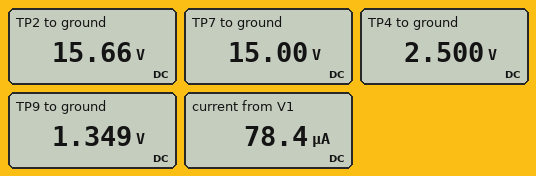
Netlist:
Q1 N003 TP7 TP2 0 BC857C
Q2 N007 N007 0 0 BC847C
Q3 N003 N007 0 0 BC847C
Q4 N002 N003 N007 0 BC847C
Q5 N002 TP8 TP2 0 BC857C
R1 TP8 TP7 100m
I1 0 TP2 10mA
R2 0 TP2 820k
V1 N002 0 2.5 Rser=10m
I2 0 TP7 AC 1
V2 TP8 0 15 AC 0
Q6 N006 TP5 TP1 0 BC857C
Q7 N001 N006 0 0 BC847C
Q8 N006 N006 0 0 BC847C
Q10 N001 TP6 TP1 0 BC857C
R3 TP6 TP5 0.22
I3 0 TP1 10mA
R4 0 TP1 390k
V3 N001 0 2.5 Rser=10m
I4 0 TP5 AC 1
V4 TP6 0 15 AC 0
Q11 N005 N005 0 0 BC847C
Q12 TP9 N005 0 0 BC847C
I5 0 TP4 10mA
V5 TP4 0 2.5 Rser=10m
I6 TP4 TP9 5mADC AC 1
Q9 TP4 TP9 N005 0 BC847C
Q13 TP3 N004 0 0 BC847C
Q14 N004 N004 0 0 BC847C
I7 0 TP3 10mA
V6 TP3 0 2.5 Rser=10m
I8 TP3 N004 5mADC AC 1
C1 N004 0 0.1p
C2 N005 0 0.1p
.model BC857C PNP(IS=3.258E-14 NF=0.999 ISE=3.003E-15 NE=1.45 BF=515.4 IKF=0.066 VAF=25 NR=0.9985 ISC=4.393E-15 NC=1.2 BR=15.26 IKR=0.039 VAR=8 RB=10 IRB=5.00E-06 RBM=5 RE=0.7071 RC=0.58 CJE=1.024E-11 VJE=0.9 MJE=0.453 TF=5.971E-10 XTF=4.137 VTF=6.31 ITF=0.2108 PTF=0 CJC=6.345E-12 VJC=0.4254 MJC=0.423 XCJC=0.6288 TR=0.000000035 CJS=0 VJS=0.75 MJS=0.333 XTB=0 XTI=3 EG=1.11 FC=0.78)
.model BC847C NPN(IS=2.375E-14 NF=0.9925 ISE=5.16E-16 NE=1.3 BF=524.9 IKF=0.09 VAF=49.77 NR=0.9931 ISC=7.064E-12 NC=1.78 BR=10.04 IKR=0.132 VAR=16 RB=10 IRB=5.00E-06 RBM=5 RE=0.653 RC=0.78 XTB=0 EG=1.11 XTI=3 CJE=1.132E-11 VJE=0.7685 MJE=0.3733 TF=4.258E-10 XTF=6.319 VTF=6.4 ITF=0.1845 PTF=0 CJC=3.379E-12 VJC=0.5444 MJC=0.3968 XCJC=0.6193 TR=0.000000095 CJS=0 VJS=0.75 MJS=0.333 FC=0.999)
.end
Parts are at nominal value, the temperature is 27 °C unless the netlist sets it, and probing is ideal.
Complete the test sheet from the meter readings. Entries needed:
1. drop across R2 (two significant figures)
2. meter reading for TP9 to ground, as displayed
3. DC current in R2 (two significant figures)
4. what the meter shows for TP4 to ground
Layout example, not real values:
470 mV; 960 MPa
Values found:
16 V; 1.349 V; 19 µA; 2.500 V
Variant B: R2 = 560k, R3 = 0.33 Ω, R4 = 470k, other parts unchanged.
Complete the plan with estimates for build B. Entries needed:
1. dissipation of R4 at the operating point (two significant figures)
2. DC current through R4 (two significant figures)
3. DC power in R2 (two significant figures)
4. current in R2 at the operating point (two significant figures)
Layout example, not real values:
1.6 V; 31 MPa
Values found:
520 µW; 33 µA; 440 µW; 28 µA
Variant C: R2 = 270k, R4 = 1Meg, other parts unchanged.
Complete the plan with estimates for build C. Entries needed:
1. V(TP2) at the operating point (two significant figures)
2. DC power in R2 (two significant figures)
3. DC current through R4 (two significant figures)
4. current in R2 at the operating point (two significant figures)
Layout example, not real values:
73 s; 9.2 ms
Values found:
16 V; 910 µW; 16 µA; 58 µA
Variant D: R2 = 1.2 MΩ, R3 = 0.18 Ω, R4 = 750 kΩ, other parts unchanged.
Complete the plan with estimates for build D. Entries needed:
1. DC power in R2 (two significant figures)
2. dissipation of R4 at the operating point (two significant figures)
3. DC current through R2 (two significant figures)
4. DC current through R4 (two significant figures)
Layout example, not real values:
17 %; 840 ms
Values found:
200 µW; 330 µW; 13 µA; 21 µA
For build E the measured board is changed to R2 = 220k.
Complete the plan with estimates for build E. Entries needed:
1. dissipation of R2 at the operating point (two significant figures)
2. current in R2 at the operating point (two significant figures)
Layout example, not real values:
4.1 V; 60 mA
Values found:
1.1 mW; 71 µA
